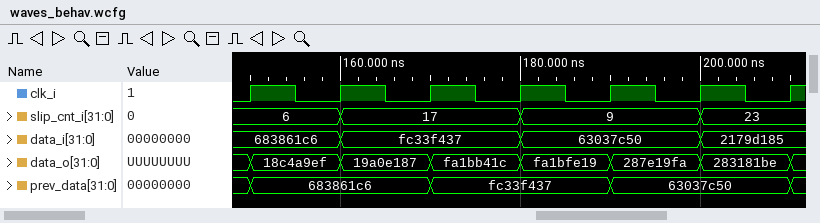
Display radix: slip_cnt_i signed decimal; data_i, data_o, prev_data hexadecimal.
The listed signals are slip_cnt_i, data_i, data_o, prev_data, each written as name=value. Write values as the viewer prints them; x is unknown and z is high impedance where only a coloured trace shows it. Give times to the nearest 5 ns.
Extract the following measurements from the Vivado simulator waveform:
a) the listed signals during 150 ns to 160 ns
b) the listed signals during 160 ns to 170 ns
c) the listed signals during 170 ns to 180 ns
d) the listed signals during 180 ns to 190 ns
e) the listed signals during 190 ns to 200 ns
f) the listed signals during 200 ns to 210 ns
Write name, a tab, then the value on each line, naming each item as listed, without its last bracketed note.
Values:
the listed signals during 150 ns to 160 ns	slip_cnt_i=6, data_i=683861c6, data_o=18c4a9ef, prev_data=683861c6
the listed signals during 160 ns to 170 ns	slip_cnt_i=17, data_i=fc33f437, data_o=19a0e187, prev_data=683861c6
the listed signals during 170 ns to 180 ns	slip_cnt_i=17, data_i=fc33f437, data_o=fa1bb41c, prev_data=fc33f437
the listed signals during 180 ns to 190 ns	slip_cnt_i=9, data_i=63037c50, data_o=fa1bfe19, prev_data=fc33f437
the listed signals during 190 ns to 200 ns	slip_cnt_i=9, data_i=63037c50, data_o=287e19fa, prev_data=63037c50
the listed signals during 200 ns to 210 ns	slip_cnt_i=23, data_i=2179d185, data_o=283181be, prev_data=63037c50
